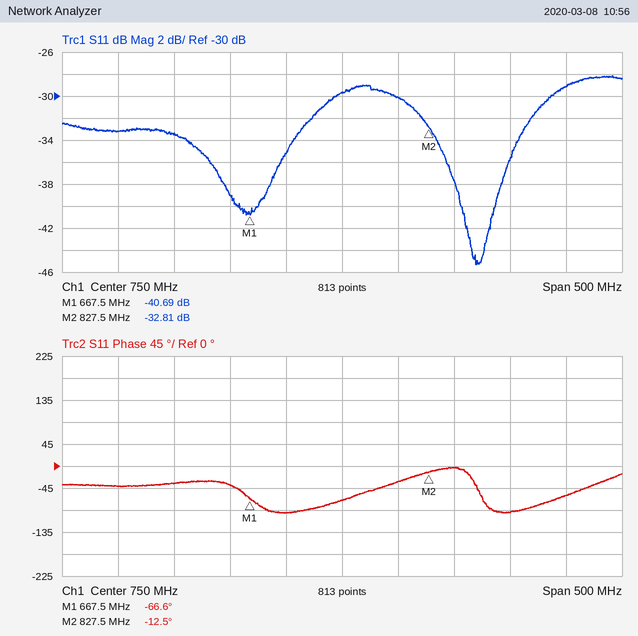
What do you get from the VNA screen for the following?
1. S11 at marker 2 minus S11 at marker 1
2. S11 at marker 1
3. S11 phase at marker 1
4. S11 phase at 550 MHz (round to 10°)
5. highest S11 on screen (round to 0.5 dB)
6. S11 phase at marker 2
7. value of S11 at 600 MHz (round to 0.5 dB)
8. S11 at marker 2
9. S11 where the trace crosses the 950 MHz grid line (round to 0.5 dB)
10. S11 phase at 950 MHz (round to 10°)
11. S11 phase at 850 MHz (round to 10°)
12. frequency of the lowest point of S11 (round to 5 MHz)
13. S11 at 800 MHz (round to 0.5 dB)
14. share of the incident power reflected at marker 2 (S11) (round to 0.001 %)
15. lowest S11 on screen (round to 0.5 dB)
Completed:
7.88 dB
-40.69 dB
-66.6°
-40°
-28.0 dB
-12.5°
-33.5 dB
-32.81 dB
-29.0 dB
-60°
0°
870 MHz
-30.0 dB
0.052 %
-45.5 dB
